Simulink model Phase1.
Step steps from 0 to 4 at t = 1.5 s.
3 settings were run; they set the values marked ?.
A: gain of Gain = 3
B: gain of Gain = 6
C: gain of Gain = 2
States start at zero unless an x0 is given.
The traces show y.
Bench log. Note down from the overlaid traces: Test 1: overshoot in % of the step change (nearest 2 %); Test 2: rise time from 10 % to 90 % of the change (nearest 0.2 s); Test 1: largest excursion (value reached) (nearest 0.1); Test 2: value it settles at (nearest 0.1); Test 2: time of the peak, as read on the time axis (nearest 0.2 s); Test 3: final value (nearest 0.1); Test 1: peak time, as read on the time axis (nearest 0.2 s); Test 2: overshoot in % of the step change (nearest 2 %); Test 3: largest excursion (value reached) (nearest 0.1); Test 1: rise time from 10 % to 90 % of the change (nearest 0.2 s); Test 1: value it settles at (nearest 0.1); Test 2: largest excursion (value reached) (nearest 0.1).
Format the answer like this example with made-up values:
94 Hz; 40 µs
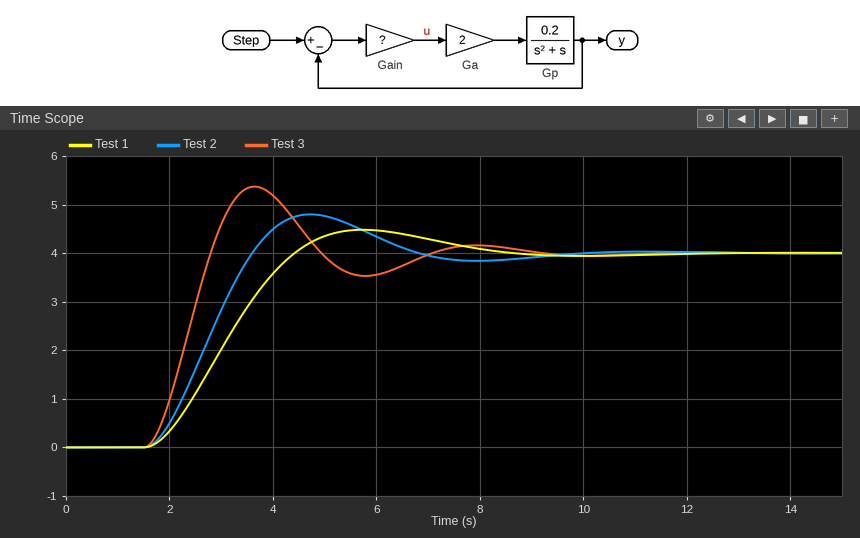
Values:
12 %; 1.4 s; 4.5; 4.0; 4.8 s; 4.0; 5.8 s; 20 %; 5.4; 2.0 s; 4.0; 4.8
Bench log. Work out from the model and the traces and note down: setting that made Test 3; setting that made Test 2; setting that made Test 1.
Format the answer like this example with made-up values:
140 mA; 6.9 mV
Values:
B; A; C
